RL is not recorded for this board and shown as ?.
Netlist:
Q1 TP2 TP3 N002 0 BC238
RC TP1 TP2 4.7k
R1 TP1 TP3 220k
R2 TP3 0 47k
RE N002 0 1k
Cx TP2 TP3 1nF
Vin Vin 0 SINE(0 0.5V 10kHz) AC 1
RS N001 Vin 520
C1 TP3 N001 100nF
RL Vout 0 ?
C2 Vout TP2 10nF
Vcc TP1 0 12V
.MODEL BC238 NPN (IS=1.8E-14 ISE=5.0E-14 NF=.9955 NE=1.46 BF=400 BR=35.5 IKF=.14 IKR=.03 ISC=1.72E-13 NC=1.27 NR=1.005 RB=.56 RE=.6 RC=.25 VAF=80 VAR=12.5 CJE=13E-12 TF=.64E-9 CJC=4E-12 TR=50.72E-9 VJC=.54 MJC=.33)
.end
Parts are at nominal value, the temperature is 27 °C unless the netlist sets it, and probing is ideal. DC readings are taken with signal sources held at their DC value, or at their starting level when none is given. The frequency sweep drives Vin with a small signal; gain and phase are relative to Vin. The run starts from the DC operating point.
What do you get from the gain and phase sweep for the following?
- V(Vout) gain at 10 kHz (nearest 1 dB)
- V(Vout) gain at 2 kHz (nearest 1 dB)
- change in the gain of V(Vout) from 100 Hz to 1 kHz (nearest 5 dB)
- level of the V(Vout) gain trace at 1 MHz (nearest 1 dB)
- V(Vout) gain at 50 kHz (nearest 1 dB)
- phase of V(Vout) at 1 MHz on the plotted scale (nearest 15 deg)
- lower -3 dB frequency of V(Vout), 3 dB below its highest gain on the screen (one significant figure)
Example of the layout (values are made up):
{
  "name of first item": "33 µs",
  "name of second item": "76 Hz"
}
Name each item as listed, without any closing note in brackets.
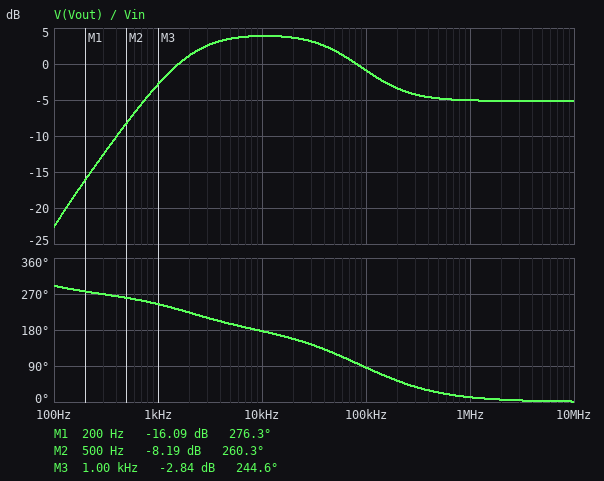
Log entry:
{
  "V(Vout) gain at 10 kHz": "4 dB",
  "V(Vout) gain at 2 kHz": "1 dB",
  "change in the gain of V(Vout) from 100 Hz to 1 kHz": "20 dB",
  "level of the V(Vout) gain trace at 1 MHz": "-5 dB",
  "V(Vout) gain at 50 kHz": "2 dB",
  "phase of V(Vout) at 1 MHz on the plotted scale": "15 deg",
  "lower -3 dB frequency of V(Vout), 3 dB below its highest gain on the screen": "2 kHz"
}
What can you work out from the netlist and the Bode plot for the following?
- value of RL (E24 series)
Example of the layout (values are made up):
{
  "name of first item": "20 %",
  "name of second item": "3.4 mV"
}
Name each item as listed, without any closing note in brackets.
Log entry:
{
  "value of RL": "3 kΩ"
}
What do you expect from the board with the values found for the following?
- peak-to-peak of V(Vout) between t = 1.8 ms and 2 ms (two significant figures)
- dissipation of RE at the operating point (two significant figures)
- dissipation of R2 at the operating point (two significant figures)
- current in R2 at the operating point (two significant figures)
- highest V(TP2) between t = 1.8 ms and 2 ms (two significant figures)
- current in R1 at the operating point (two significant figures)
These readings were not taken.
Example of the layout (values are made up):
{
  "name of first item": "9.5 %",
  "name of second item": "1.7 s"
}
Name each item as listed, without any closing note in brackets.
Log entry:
{
  "peak-to-peak of V(Vout) between t = 1.8 ms and 2 ms": "1.6 V",
  "dissipation of RE at the operating point": "1.7 mW",
  "dissipation of R2 at the operating point": "80 µW",
  "current in R2 at the operating point": "41 µA",
  "highest V(TP2) between t = 1.8 ms and 2 ms": "6.8 V",
  "current in R1 at the operating point": "46 µA"
}
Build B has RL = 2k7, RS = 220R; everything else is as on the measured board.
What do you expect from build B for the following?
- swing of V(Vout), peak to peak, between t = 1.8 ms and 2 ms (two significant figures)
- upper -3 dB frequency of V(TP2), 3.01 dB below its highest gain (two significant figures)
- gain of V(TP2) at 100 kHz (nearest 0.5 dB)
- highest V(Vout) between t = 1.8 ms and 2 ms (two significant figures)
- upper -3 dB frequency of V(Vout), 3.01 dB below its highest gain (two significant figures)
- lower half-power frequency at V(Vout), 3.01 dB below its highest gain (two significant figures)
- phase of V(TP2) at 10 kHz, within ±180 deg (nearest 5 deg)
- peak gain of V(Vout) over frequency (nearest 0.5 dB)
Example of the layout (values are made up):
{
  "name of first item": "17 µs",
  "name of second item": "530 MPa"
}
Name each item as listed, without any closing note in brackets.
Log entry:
{
  "swing of V(Vout), peak to peak, between t = 1.8 ms and 2 ms": "1.5 V",
  "upper -3 dB frequency of V(TP2), 3.01 dB below its highest gain": "2.6 kHz",
  "gain of V(TP2) at 100 kHz": "1.0 dB",
  "highest V(Vout) between t = 1.8 ms and 2 ms": "750 mV",
  "upper -3 dB frequency of V(Vout), 3.01 dB below its highest gain": "110 kHz",
  "lower half-power frequency at V(Vout), 3.01 dB below its highest gain": "2.0 kHz",
  "phase of V(TP2) at 10 kHz, within ±180 deg": "150 deg",
  "peak gain of V(Vout) over frequency": "3.5 dB"
}
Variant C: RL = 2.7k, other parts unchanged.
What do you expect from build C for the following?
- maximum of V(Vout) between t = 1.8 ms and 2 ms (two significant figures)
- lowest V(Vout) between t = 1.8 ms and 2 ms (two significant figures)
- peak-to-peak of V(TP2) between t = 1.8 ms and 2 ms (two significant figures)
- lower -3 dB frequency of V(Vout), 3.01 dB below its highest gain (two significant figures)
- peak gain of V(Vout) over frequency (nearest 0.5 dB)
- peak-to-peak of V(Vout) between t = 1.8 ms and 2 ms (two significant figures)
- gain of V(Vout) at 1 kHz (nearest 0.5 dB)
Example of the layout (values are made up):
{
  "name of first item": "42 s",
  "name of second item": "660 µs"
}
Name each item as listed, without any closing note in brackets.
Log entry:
{
  "maximum of V(Vout) between t = 1.8 ms and 2 ms": "730 mV",
  "lowest V(Vout) between t = 1.8 ms and 2 ms": "-730 mV",
  "peak-to-peak of V(TP2) between t = 1.8 ms and 2 ms": "1.7 V",
  "lower -3 dB frequency of V(Vout), 3.01 dB below its highest gain": "2.0 kHz",
  "peak gain of V(Vout) over frequency": "3.5 dB",
  "peak-to-peak of V(Vout) between t = 1.8 ms and 2 ms": "1.5 V",
  "gain of V(Vout) at 1 kHz": "-3.5 dB"
}
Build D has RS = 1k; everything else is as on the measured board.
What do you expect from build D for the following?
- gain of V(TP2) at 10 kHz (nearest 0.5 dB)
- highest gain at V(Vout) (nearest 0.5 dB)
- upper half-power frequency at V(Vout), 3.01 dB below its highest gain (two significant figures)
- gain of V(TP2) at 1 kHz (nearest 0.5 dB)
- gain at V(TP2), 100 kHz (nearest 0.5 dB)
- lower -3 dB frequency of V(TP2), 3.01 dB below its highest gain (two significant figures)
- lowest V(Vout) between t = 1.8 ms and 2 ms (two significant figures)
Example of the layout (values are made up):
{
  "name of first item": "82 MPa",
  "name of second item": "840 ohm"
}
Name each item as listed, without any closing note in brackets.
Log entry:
{
  "gain of V(TP2) at 10 kHz": "4.5 dB",
  "highest gain at V(Vout)": "3.5 dB",
  "upper half-power frequency at V(Vout), 3.01 dB below its highest gain": "45 kHz",
  "gain of V(TP2) at 1 kHz": "11.5 dB",
  "gain at V(TP2), 100 kHz": "-3.5 dB",
  "lower -3 dB frequency of V(TP2), 3.01 dB below its highest gain": "41 Hz",
  "lowest V(Vout) between t = 1.8 ms and 2 ms": "-750 mV"
}
